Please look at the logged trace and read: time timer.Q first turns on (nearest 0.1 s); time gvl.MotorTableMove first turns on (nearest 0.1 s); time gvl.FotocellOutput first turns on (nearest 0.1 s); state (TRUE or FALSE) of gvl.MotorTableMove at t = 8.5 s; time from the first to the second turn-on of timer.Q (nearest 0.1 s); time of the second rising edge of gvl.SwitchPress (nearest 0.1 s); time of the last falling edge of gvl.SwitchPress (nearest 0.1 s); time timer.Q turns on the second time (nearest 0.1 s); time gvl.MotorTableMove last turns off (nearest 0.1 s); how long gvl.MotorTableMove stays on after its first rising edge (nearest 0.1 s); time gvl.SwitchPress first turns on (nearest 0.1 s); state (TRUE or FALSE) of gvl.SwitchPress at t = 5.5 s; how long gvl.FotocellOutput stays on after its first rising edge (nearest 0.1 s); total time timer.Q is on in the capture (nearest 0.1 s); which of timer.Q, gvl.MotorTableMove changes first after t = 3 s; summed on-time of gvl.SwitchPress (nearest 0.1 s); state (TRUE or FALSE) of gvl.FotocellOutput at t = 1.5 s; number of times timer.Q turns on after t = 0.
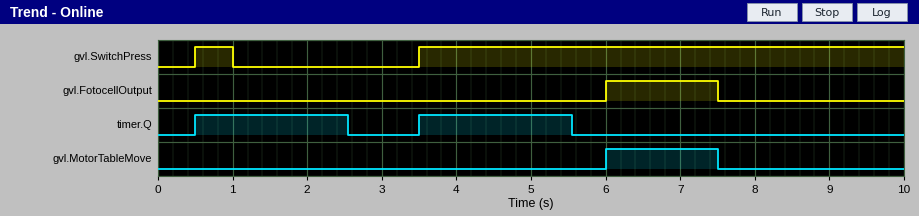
0.5 s
6.0 s
6.0 s
FALSE
3.0 s
3.5 s
1.0 s
3.5 s
7.5 s
1.5 s
0.5 s
TRUE
1.5 s
4.1 s
timer.Q
7.0 s
FALSE
2
